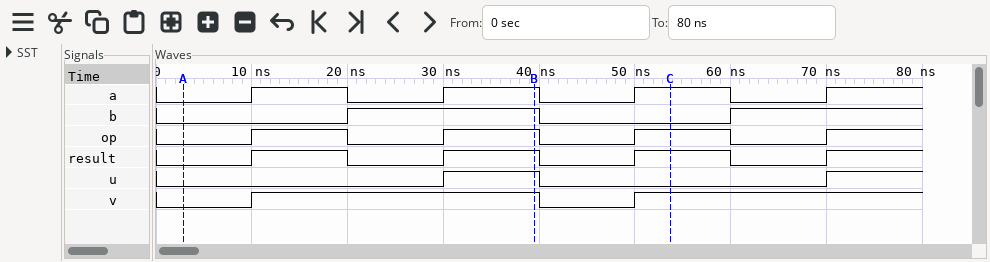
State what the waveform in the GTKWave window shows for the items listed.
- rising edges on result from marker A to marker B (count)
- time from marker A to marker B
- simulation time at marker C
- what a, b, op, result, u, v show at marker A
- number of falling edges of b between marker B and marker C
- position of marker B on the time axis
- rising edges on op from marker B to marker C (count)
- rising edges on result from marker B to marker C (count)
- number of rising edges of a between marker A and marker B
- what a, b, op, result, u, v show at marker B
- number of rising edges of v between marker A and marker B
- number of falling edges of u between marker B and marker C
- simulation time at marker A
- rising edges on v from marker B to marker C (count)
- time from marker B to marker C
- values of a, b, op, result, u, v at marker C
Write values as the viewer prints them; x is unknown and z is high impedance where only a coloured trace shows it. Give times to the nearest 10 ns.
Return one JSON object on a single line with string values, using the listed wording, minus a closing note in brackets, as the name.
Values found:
{"rising edges on result from marker A to marker B": "2", "time from marker A to marker B": "40 ns", "simulation time at marker C": "50 ns", "what a, b, op, result, u, v show at marker A": "a=0, b=0, op=0, result=0, u=0, v=0", "number of falling edges of b between marker B and marker C": "1", "position of marker B on the time axis": "40 ns", "rising edges on op from marker B to marker C": "1", "rising edges on result from marker B to marker C": "1", "number of rising edges of a between marker A and marker B": "2", "what a, b, op, result, u, v show at marker B": "a=1, b=1, op=1, result=1, u=1, v=1", "number of rising edges of v between marker A and marker B": "1", "number of falling edges of u between marker B and marker C": "1", "simulation time at marker A": "0 ns", "rising edges on v from marker B to marker C": "1", "time from marker B to marker C": "10 ns", "values of a, b, op, result, u, v at marker C": "a=1, b=0, op=1, result=1, u=0, v=1"}
